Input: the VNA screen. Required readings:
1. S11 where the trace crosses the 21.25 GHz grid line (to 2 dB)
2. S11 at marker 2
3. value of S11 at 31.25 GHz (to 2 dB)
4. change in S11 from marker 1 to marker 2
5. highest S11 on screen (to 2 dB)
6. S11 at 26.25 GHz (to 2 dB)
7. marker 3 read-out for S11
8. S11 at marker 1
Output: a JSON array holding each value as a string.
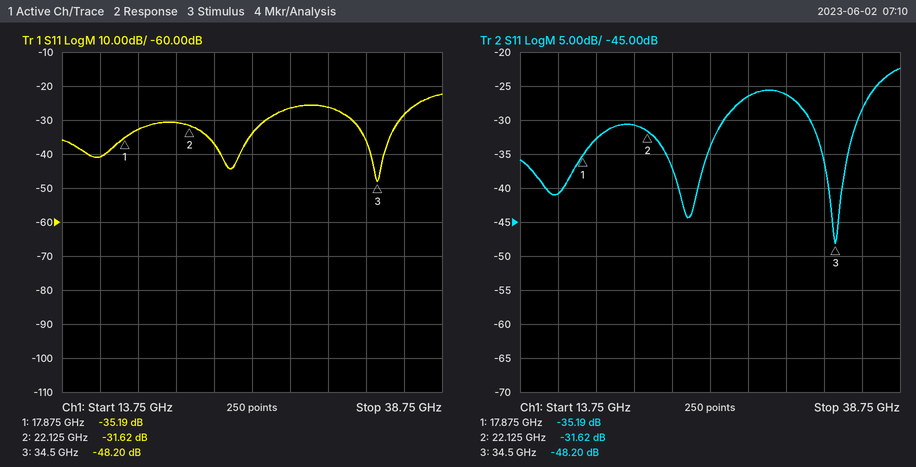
["-30 dB", "-31.62 dB", "-26 dB", "3.57 dB", "-22 dB", "-34 dB", "-48.20 dB", "-35.19 dB"]
